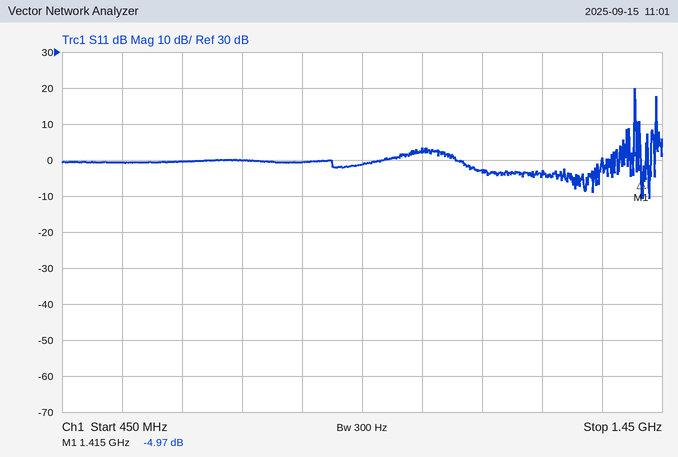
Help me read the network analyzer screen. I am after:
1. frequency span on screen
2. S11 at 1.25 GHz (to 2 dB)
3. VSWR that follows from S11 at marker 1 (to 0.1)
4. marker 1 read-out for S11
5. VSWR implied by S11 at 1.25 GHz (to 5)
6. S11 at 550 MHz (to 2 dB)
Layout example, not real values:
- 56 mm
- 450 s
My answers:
- 1 GHz
- -4 dB
- 3.6
- -4.97 dB
- 5
- 0 dB
